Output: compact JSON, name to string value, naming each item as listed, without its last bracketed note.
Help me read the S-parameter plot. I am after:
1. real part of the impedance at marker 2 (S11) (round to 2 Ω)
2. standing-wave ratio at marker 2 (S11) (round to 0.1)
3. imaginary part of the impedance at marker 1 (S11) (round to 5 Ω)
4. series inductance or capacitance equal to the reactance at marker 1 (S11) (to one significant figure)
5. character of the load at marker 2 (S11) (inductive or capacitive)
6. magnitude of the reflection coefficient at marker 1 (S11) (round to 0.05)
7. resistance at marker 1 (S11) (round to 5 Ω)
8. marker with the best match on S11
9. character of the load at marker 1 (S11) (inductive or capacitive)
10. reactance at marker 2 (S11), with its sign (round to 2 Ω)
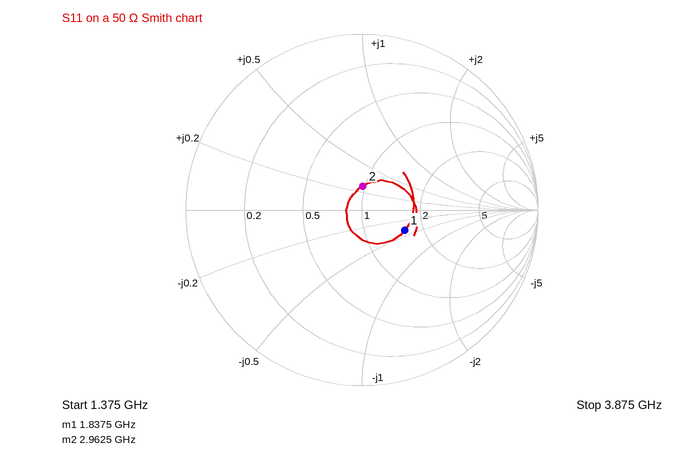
{"real part of the impedance at marker 2 (S11)": "48 Ω", "standing-wave ratio at marker 2 (S11)": "1.3", "imaginary part of the impedance at marker 1 (S11)": "-20 Ω", "series inductance or capacitance equal to the reactance at marker 1 (S11)": "4 pF", "character of the load at marker 2 (S11)": "inductive", "magnitude of the reflection coefficient at marker 1 (S11)": "0.25", "resistance at marker 1 (S11)": "80 Ω", "marker with the best match on S11": "marker 2", "character of the load at marker 1 (S11)": "capacitive", "reactance at marker 2 (S11), with its sign": "+14 Ω"}
